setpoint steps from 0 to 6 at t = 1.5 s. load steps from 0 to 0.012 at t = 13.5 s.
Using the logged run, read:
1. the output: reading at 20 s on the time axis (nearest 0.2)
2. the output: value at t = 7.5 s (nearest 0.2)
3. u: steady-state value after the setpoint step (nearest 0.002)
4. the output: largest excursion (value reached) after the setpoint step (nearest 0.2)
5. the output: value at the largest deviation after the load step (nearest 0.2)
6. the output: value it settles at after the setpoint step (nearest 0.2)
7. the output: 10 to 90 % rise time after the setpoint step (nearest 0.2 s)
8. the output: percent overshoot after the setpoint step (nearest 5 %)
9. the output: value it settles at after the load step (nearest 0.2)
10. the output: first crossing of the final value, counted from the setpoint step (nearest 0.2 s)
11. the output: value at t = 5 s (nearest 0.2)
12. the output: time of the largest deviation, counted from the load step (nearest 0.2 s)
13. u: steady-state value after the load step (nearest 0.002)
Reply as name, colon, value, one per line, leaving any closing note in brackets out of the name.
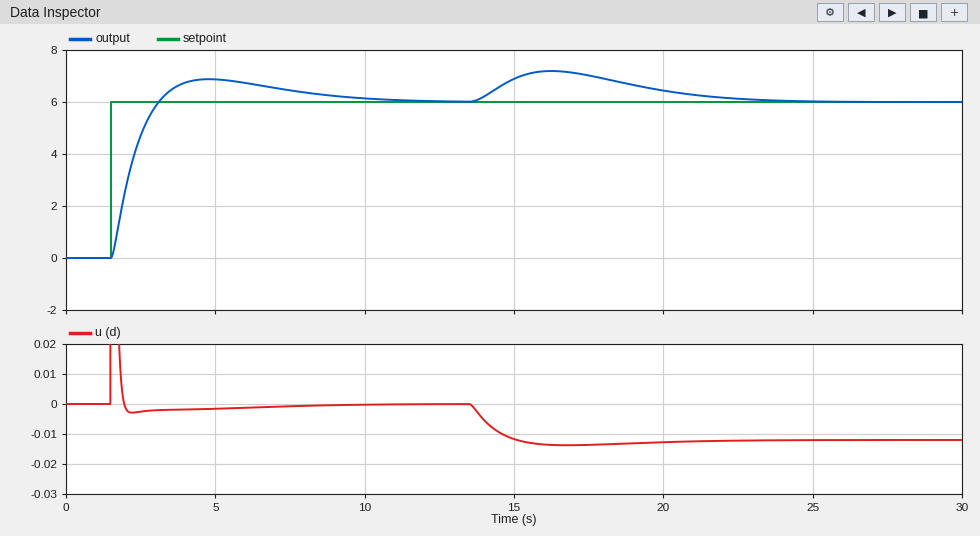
the output: reading at 20 s on the time axis: 6.4
the output: value at t = 7.5 s: 6.4
u: steady-state value after the setpoint step: 0.000
the output: largest excursion (value reached) after the setpoint step: 6.8
the output: value at the largest deviation after the load step: 7.2
the output: value it settles at after the setpoint step: 6.0
the output: 10 to 90 % rise time after the setpoint step: 1.2 s
the output: percent overshoot after the setpoint step: 15 %
the output: value it settles at after the load step: 6.0
the output: first crossing of the final value, counted from the setpoint step: 1.6 s
the output: value at t = 5 s: 6.8
the output: time of the largest deviation, counted from the load step: 2.8 s
u: steady-state value after the load step: -0.012
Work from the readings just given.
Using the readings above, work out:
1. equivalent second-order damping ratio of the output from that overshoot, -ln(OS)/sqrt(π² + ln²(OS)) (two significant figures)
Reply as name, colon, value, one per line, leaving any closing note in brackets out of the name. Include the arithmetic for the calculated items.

equivalent second-order damping ratio of the output from that overshoot, -ln(OS)/sqrt(π² + ln²(OS)): ln(0.15) = -1.897; 1.897 / sqrt(9.870 + 3.599) = 0.52
